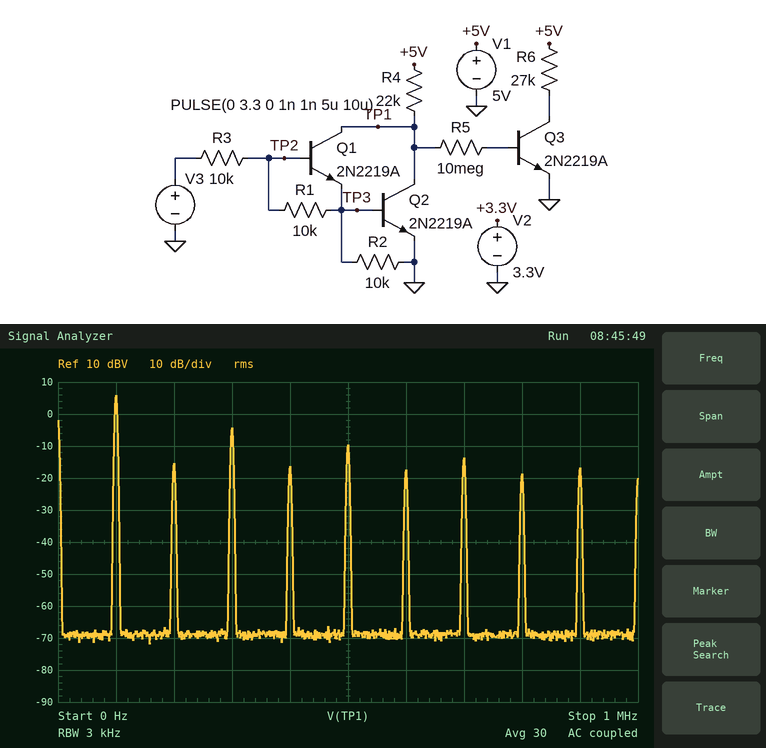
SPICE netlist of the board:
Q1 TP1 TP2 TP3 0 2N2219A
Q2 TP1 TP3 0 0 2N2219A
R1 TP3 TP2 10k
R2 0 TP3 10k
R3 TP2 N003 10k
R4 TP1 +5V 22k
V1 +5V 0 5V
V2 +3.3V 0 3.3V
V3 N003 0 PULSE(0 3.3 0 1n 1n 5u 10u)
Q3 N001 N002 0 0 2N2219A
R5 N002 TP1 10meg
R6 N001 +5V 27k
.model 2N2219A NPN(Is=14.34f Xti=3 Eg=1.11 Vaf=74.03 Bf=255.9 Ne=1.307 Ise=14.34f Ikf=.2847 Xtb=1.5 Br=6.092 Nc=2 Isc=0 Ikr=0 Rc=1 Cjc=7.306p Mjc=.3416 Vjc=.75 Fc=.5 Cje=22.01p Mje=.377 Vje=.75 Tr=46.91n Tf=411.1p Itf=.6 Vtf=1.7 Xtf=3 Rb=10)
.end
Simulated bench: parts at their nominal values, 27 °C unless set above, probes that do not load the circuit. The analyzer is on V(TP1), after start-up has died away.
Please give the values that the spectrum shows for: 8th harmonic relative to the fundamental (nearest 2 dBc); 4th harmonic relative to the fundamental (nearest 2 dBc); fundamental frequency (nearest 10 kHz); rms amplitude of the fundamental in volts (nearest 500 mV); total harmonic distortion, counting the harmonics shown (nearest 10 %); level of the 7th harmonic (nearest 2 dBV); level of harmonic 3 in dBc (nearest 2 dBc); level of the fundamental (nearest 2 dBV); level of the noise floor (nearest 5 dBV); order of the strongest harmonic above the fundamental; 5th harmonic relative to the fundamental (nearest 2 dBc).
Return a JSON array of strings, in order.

["-24 dBc", "-22 dBc", "100 kHz", "2.0 V", "40 %", "-14 dBV", "-10 dBc", "6 dBV", "-70 dBV", "3", "-16 dBc"]
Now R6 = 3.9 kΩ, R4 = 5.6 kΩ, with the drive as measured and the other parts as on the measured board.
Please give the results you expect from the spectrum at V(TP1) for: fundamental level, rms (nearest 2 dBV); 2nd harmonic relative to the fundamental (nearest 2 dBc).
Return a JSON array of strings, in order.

["6 dBV", "-24 dBc"]
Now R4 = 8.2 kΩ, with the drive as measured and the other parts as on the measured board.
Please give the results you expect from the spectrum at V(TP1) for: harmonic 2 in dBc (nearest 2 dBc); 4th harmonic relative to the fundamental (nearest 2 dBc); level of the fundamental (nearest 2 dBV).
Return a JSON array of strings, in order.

["-24 dBc", "-24 dBc", "6 dBV"]
